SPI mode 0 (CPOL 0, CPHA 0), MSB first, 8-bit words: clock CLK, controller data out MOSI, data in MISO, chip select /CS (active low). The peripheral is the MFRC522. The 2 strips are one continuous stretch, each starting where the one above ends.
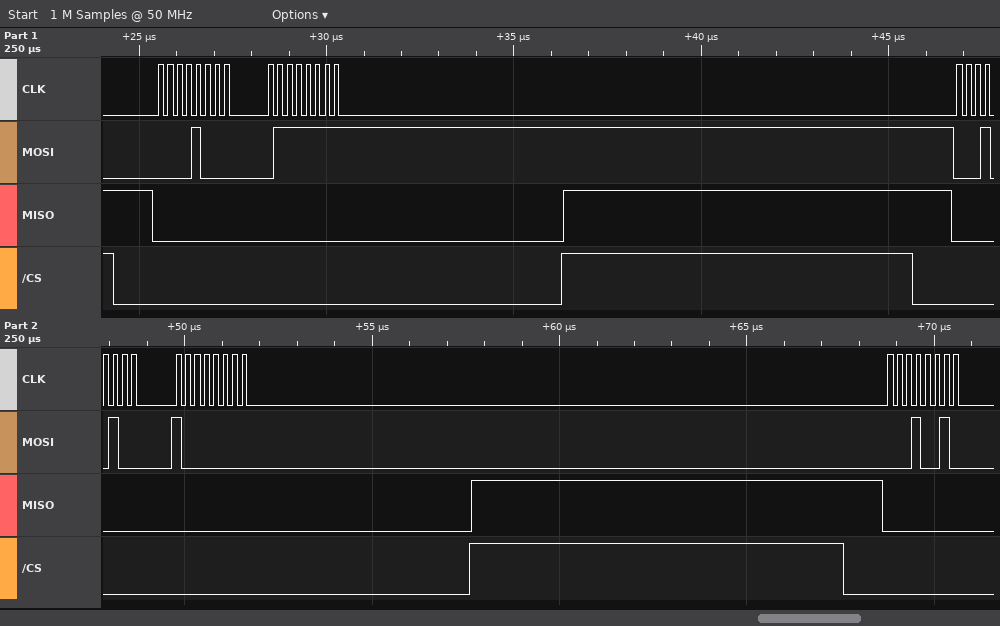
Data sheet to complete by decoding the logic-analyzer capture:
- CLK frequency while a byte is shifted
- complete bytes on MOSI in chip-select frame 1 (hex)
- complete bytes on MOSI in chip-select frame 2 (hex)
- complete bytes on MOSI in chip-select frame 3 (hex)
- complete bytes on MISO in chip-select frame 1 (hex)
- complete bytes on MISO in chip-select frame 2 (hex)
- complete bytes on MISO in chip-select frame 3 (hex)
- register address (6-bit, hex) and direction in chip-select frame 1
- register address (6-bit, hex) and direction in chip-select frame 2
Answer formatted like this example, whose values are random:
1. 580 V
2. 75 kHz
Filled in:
1. 4 MHz
2. 0x08 0x7F
3. 0x14 0x80
4. 0x12
5. 0x00 0x00
6. 0x00 0x00
7. 0x00
8. 0x04 write
9. 0x0A write
